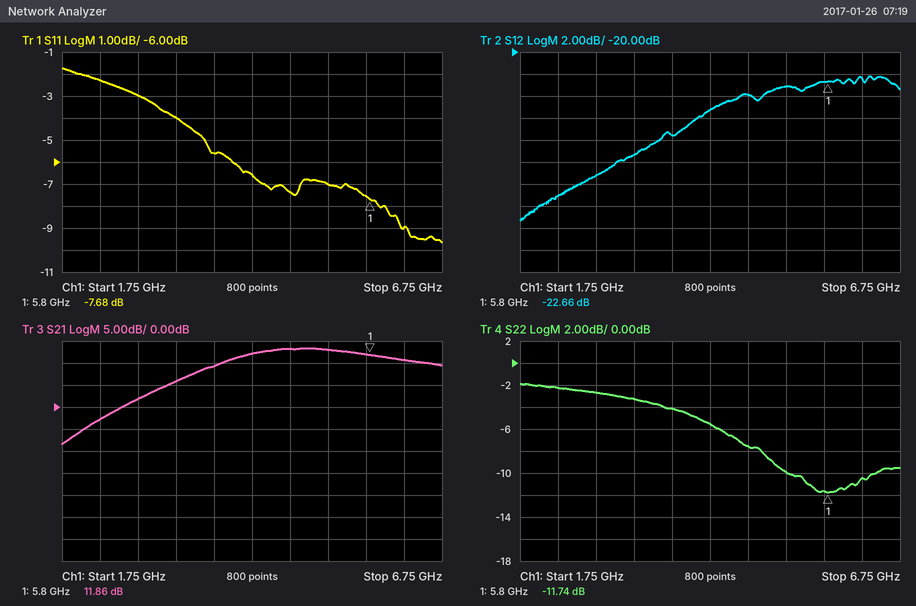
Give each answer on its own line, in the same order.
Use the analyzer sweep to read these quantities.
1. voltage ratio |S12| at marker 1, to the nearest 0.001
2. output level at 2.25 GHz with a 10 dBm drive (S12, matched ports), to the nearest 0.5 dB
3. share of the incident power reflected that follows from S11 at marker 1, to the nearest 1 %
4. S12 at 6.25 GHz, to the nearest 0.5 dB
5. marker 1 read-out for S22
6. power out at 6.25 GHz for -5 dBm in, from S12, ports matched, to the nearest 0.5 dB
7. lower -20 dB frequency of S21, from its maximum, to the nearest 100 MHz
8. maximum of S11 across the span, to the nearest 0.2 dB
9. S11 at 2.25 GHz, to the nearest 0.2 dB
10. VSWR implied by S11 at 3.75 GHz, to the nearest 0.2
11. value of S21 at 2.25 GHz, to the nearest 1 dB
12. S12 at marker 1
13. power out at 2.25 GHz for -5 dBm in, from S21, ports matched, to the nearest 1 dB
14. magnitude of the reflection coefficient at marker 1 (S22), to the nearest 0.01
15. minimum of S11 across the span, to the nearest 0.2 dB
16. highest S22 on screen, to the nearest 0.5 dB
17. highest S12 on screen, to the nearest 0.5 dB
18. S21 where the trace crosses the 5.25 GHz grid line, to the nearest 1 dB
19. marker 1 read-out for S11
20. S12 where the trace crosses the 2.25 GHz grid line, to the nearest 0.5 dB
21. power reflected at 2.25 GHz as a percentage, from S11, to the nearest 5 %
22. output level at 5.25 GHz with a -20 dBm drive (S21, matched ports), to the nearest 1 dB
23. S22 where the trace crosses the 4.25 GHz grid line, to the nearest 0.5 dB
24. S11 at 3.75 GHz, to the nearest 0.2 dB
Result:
0.074
-23.0 dBm
17 %
-22.5 dB
-11.74 dB
-27.5 dBm
1.9 GHz
-1.8 dB
-2.2 dB
3.2
-3 dB
-22.66 dB
-8 dBm
0.26
-9.6 dB
-2.0 dB
-22.0 dB
13 dB
-7.68 dB
-33.0 dB
60 %
-7 dBm
-5.5 dB
-5.6 dB
